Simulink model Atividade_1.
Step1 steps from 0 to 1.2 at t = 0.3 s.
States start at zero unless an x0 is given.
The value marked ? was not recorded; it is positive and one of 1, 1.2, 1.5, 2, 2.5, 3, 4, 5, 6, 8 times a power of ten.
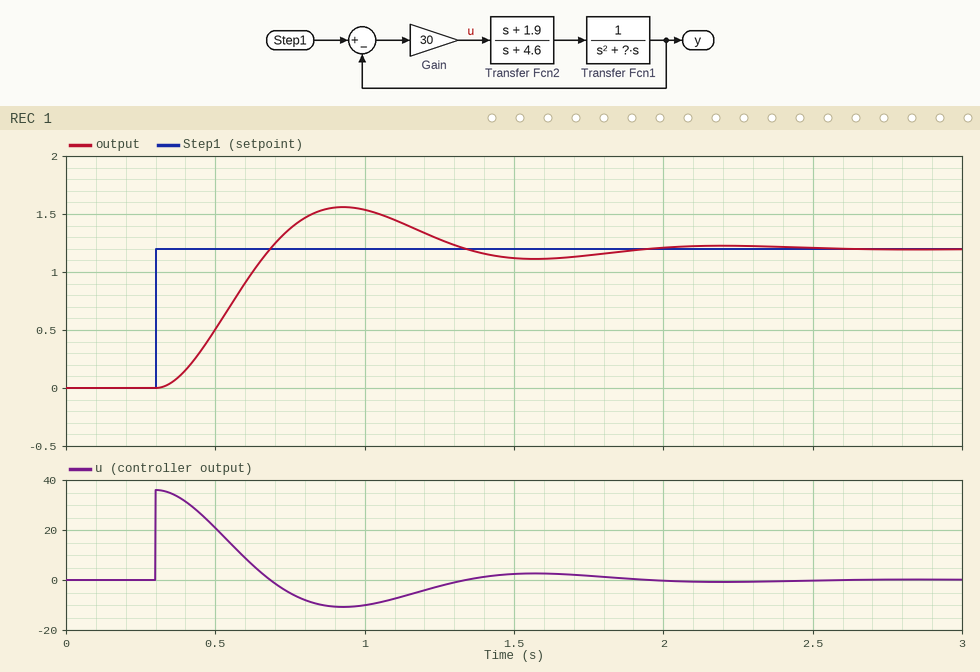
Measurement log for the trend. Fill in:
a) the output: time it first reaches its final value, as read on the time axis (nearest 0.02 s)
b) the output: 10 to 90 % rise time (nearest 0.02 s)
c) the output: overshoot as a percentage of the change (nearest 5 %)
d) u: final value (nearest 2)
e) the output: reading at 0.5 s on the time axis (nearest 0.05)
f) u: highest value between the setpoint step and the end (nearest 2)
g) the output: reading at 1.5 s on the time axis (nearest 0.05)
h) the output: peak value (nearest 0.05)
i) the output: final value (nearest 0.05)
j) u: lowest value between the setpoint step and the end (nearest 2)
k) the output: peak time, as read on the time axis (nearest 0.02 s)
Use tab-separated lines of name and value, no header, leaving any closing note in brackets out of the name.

the output: time it first reaches its final value, as read on the time axis	0.68 s
the output: 10 to 90 % rise time	0.26 s
the output: overshoot as a percentage of the change	30 %
u: final value	0
the output: reading at 0.5 s on the time axis	0.50
u: highest value between the setpoint step and the end	36
the output: reading at 1.5 s on the time axis	1.10
the output: peak value	1.55
the output: final value	1.20
u: lowest value between the setpoint step and the end	-10
the output: peak time, as read on the time axis	0.92 s
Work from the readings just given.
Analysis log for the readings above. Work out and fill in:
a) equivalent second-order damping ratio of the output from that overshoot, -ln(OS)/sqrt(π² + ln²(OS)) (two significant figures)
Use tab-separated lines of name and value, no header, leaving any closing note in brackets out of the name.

equivalent second-order damping ratio of the output from that overshoot, -ln(OS)/sqrt(π² + ln²(OS))	0.36
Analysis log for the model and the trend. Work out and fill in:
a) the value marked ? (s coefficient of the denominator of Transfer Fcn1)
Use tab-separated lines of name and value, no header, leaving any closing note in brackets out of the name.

the value marked ?	1.5
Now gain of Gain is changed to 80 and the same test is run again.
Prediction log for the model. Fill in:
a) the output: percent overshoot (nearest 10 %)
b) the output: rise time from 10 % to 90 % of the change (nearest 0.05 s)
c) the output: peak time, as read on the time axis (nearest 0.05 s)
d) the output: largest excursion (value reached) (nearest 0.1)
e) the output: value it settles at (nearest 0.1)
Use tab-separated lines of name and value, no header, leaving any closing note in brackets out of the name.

the output: percent overshoot	50 %
the output: rise time from 10 % to 90 % of the change	0.15 s
the output: peak time, as read on the time axis	0.65 s
the output: largest excursion (value reached)	1.8
the output: value it settles at	1.2
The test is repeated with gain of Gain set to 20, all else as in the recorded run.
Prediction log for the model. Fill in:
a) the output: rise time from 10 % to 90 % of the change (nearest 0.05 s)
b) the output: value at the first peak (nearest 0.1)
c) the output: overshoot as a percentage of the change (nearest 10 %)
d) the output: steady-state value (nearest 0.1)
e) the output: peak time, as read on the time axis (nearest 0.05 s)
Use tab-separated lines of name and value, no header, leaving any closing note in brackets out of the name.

the output: rise time from 10 % to 90 % of the change	0.35 s
the output: value at the first peak	1.5
the output: overshoot as a percentage of the change	20 %
the output: steady-state value	1.2
the output: peak time, as read on the time axis	1.10 s
